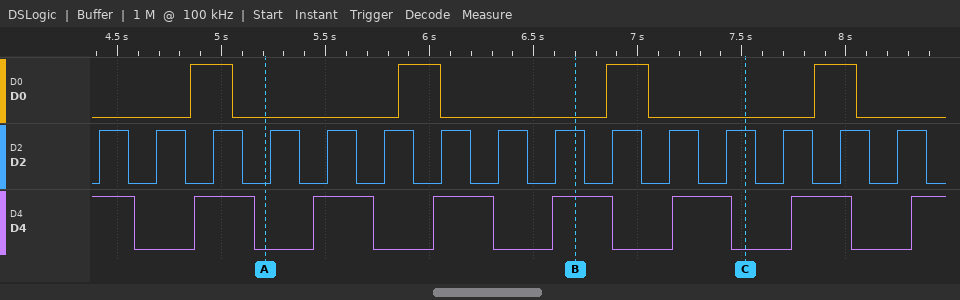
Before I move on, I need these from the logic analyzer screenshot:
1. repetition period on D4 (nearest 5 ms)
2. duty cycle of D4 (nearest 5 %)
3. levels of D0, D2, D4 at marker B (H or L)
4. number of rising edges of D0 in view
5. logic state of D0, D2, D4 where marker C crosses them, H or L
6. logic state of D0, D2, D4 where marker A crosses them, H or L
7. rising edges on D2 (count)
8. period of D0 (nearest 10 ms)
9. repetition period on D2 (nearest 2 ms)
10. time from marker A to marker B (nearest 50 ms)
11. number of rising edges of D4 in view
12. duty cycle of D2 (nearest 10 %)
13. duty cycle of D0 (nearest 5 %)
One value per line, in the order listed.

575 ms
50 %
D0=L, D2=H, D4=H
4
D0=L, D2=H, D4=L
D0=L, D2=L, D4=L
15
1000 ms
274 ms
1500 ms
7
50 %
20 %
